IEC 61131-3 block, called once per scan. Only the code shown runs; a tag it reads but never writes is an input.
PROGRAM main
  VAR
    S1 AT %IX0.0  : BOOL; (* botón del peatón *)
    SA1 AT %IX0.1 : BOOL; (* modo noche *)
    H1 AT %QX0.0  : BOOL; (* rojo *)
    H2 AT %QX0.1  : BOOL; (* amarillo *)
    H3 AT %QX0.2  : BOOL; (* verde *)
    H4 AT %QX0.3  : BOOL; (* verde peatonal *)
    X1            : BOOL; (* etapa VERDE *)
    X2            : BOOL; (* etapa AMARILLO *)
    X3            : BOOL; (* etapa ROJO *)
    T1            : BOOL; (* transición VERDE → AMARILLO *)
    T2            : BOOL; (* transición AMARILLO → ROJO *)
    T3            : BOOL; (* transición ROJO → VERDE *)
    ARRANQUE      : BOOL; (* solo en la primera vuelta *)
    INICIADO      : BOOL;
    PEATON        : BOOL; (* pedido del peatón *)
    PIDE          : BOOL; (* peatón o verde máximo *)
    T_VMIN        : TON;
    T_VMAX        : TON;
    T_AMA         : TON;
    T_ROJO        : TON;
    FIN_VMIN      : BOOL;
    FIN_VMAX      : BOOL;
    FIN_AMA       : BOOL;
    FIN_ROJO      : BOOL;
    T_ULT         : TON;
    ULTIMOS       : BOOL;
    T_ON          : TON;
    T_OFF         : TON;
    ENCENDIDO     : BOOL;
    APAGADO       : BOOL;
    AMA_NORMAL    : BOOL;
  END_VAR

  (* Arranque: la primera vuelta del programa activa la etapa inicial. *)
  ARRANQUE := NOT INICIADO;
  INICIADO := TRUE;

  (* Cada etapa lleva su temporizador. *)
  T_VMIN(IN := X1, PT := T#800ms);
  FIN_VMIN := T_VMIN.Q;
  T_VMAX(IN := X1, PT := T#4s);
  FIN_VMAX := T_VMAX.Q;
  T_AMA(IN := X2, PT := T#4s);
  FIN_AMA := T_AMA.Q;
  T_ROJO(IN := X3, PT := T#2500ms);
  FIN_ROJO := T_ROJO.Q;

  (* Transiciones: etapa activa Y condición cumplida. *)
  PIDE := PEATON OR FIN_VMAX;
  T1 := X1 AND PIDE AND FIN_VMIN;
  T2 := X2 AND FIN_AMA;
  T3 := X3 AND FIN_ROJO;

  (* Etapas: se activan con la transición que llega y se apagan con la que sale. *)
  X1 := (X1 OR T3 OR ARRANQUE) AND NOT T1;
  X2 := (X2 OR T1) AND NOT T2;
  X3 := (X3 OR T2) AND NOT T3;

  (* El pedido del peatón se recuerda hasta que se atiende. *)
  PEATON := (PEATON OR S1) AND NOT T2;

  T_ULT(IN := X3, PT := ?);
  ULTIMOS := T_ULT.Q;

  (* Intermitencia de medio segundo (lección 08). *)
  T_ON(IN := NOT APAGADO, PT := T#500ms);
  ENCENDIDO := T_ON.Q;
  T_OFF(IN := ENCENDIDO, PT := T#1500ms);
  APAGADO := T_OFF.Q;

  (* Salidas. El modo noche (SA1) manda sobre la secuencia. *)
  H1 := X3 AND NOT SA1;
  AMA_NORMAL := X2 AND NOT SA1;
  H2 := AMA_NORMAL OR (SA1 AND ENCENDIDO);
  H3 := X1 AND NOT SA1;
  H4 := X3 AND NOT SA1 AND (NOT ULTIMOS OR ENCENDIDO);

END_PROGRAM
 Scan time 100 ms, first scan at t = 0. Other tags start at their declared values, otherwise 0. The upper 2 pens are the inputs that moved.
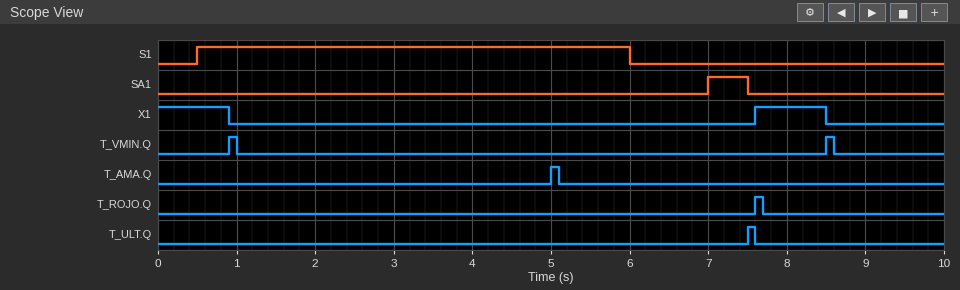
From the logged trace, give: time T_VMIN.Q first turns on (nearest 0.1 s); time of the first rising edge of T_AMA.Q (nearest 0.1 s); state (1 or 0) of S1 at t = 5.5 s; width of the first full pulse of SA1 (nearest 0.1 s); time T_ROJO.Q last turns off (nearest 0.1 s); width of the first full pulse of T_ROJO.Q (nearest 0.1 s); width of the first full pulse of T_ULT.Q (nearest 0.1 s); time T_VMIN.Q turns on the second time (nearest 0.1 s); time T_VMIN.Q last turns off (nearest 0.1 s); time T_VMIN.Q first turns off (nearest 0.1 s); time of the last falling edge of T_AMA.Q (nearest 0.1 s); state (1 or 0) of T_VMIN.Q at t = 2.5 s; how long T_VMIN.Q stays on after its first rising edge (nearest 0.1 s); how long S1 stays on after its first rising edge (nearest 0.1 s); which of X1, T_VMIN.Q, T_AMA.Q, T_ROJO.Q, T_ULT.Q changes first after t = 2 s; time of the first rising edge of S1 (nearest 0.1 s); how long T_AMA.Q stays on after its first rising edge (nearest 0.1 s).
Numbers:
0.9 s
5.0 s
1
0.5 s
7.7 s
0.1 s
0.1 s
8.5 s
8.6 s
1.0 s
5.1 s
0
0.1 s
5.5 s
T_AMA.Q
0.5 s
0.1 s
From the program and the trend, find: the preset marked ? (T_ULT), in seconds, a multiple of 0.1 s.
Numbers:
2.5 s
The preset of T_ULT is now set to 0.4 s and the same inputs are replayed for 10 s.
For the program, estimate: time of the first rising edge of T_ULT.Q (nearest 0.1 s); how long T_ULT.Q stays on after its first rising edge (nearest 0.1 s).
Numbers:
5.4 s
2.2 s
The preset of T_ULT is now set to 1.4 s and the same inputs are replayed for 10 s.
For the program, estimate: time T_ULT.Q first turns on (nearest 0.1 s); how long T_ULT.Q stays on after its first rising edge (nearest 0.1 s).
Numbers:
6.4 s
1.2 s
